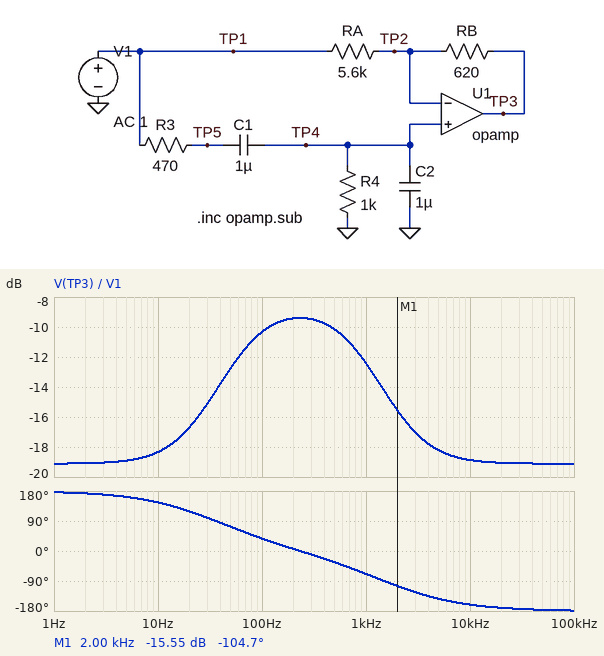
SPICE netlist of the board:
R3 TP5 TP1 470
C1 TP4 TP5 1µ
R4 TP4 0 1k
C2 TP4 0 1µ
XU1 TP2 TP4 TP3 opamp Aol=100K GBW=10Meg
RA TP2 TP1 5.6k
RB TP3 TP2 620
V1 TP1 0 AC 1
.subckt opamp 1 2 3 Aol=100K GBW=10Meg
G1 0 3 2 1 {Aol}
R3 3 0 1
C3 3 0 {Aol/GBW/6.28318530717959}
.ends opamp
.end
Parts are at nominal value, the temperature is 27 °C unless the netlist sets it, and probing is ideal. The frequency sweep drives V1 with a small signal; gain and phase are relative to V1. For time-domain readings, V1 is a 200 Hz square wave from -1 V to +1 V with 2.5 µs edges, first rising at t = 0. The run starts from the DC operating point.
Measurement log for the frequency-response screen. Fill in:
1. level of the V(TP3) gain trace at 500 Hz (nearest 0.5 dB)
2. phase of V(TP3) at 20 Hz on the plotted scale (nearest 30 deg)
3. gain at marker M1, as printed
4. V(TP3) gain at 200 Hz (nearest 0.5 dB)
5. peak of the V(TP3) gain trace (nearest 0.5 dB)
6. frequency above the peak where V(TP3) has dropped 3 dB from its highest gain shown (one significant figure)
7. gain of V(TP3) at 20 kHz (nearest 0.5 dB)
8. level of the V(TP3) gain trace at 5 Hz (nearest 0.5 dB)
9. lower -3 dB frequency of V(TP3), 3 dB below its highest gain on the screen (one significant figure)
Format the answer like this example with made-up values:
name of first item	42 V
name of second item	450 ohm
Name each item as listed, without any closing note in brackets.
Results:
level of the V(TP3) gain trace at 500 Hz	-10.0 dB
phase of V(TP3) at 20 Hz on the plotted scale	120 deg
gain at marker M1, as printed	-15.55 dB
V(TP3) gain at 200 Hz	-9.5 dB
peak of the V(TP3) gain trace	-9.5 dB
frequency above the peak where V(TP3) has dropped 3 dB from its highest gain shown	1 kHz
gain of V(TP3) at 20 kHz	-19.0 dB
level of the V(TP3) gain trace at 5 Hz	-19.0 dB
lower -3 dB frequency of V(TP3), 3 dB below its highest gain on the screen	50 Hz
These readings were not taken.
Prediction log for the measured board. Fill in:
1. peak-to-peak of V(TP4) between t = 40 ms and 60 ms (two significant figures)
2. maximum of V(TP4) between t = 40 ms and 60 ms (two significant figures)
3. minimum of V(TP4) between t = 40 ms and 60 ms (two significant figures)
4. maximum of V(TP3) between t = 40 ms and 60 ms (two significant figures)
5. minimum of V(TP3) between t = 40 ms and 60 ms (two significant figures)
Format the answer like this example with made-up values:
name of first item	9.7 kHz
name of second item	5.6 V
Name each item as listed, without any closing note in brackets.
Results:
peak-to-peak of V(TP4) between t = 40 ms and 60 ms	1.0 V
maximum of V(TP4) between t = 40 ms and 60 ms	510 mV
minimum of V(TP4) between t = 40 ms and 60 ms	-510 mV
maximum of V(TP3) between t = 40 ms and 60 ms	450 mV
minimum of V(TP3) between t = 40 ms and 60 ms	-450 mV
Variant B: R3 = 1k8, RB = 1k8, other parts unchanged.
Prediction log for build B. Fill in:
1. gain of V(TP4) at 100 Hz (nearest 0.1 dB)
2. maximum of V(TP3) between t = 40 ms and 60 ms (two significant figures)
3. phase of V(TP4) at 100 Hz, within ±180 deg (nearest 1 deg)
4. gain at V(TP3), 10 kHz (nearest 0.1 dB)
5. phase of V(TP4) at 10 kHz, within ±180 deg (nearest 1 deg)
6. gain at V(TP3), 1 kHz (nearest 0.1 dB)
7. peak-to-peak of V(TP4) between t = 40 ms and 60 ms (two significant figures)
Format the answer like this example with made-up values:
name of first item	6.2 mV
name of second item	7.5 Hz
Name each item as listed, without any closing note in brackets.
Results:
gain of V(TP4) at 100 Hz	-11.7 dB
maximum of V(TP3) between t = 40 ms and 60 ms	620 mV
phase of V(TP4) at 100 Hz, within ±180 deg	7 deg
gain at V(TP3), 10 kHz	-9.9 dB
phase of V(TP4) at 10 kHz, within ±180 deg	-88 deg
gain at V(TP3), 1 kHz	-10.3 dB
peak-to-peak of V(TP4) between t = 40 ms and 60 ms	540 mV
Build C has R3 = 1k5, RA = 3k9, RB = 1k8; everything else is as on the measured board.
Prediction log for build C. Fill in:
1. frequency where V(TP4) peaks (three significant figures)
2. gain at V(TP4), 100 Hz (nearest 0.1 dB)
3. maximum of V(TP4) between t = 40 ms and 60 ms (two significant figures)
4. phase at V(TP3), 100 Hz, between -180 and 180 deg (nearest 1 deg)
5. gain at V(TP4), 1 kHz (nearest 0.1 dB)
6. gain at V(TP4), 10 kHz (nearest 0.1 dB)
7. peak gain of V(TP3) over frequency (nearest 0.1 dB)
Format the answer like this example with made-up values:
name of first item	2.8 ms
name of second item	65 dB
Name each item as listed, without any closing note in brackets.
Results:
frequency where V(TP4) peaks	130 Hz
gain at V(TP4), 100 Hz	-11.0 dB
maximum of V(TP4) between t = 40 ms and 60 ms	300 mV
phase at V(TP3), 100 Hz, between -180 and 180 deg	128 deg
gain at V(TP4), 1 kHz	-19.9 dB
gain at V(TP4), 10 kHz	-39.5 dB
peak gain of V(TP3) over frequency	-6.7 dB
